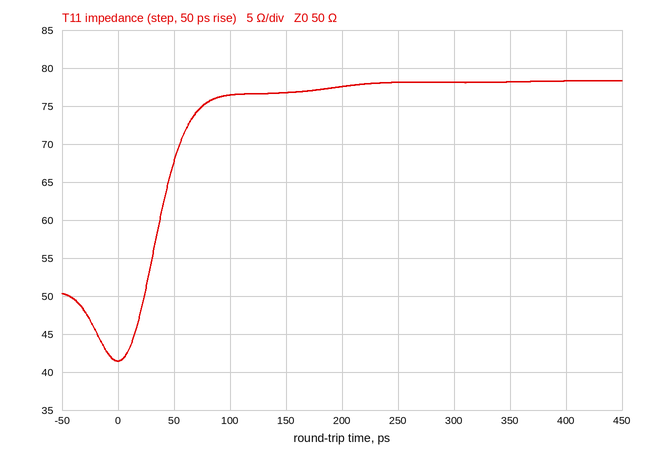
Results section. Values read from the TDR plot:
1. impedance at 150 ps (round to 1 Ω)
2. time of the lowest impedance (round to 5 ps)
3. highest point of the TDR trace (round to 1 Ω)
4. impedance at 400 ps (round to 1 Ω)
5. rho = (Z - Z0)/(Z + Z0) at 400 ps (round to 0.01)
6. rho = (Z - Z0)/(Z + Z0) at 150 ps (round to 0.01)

77 Ω
0 ps
78 Ω
78 Ω
+0.22
+0.21
